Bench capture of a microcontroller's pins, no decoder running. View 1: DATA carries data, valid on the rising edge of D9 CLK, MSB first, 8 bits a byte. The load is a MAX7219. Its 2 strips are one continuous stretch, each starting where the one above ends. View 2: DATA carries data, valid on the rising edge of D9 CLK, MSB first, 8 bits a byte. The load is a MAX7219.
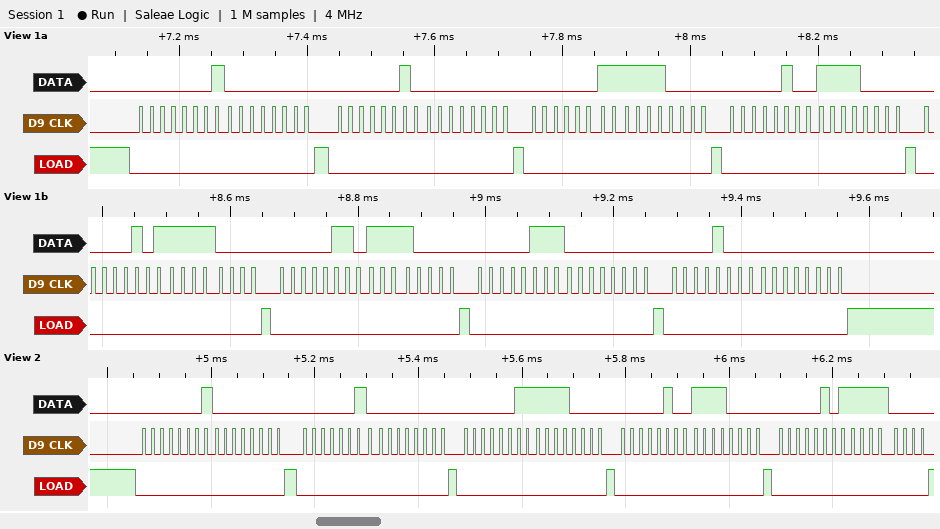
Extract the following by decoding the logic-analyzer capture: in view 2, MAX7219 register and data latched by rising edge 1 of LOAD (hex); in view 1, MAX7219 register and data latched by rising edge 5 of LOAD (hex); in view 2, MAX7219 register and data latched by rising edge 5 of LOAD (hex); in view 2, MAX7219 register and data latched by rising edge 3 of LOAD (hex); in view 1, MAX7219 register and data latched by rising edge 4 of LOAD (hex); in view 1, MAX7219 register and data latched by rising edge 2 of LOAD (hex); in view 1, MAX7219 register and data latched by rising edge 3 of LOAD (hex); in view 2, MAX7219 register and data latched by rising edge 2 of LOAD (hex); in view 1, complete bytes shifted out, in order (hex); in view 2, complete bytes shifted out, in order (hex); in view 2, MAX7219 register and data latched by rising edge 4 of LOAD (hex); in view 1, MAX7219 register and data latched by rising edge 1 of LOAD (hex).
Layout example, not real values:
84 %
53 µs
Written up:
register 0x1, data 0x00
register 0x5, data 0xF0
register 0x5, data 0xF0
register 0x3, data 0xF0
register 0x4, data 0xF0
register 0x2, data 0x00
register 0x3, data 0xF0
register 0x2, data 0x00
01 00 02 00 03 F0 04 F0 05 F0 06 F0 07 00 08 00
01 00 02 00 03 F0 04 F0 05 F0
register 0x4, data 0xF0
register 0x1, data 0x00
